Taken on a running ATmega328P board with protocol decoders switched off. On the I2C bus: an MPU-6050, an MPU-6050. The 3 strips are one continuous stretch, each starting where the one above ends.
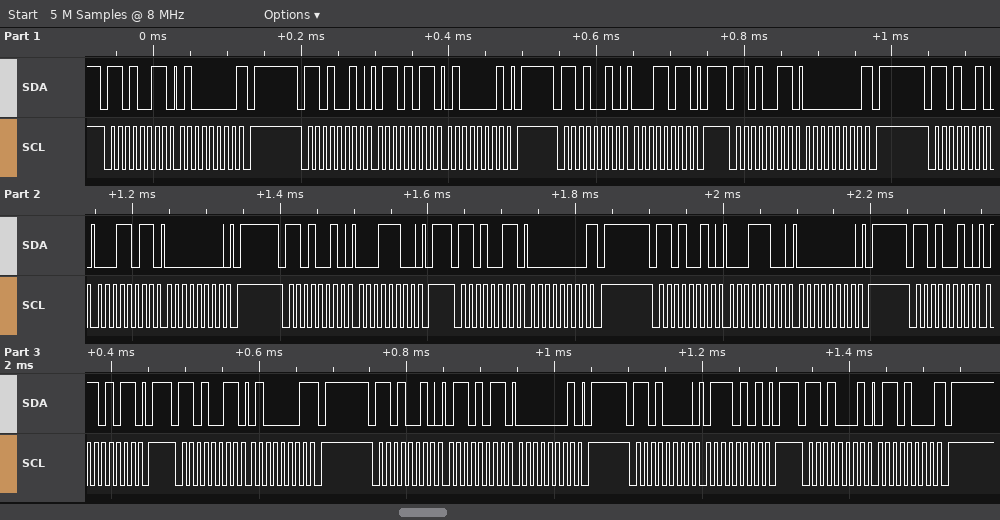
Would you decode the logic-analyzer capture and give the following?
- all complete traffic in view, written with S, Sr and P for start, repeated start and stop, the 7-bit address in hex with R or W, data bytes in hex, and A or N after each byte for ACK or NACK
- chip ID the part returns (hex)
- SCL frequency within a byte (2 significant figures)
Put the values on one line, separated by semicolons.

S 69R A 40 N P S 69W A 6B A 41 A P S 69W A 1B A P S 69R A 00 N P S 69W A 1B A 00 A P S 69W A 1C A P S 69R A 00 N P S 69W A 1C A 00 A P S 69W A 6B A P S 69R A 41 N P S 69W A 6B A 01 A P S 68W A 75 A P S 68R A 68 N P; 0x68; 100 kHz
